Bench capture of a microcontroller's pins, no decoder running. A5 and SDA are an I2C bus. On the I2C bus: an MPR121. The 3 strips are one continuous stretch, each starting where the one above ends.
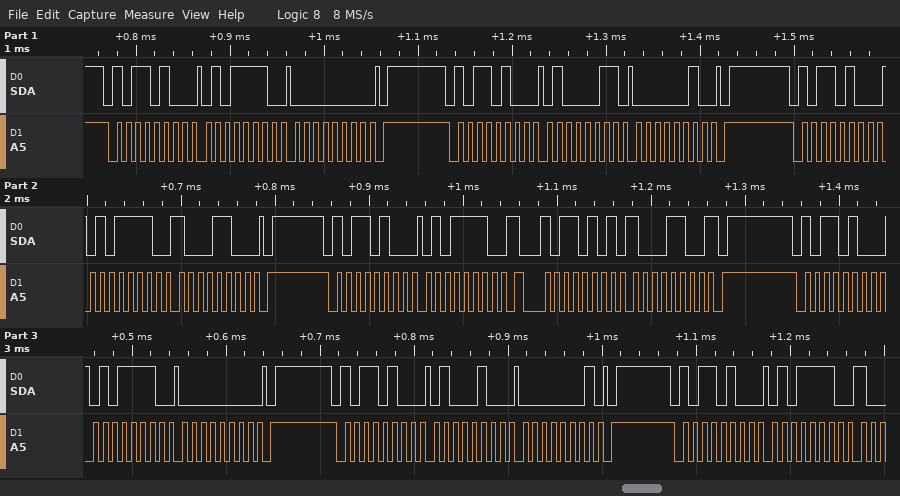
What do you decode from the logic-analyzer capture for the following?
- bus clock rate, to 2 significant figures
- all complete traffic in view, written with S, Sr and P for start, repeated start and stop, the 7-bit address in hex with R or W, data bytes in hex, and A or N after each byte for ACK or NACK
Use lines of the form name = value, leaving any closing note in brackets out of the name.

bus clock rate, to 2 significant figures = 100 kHz
all complete traffic in view, written with S, Sr and P for start, repeated start and stop, the 7-bit address in hex with R or W, data bytes in hex, and A or N after each byte for ACK or NACK = S 5AW A 5E A 00 A P S 5AW A 43 A 02 A P S 5AW A 5E A 8C A P S 5AW A 5E A Sr 5AR A 8C N P S 5AW A 5E A 00 A P S 5AW A 44 A 01 A P S 5AW A 5E A
